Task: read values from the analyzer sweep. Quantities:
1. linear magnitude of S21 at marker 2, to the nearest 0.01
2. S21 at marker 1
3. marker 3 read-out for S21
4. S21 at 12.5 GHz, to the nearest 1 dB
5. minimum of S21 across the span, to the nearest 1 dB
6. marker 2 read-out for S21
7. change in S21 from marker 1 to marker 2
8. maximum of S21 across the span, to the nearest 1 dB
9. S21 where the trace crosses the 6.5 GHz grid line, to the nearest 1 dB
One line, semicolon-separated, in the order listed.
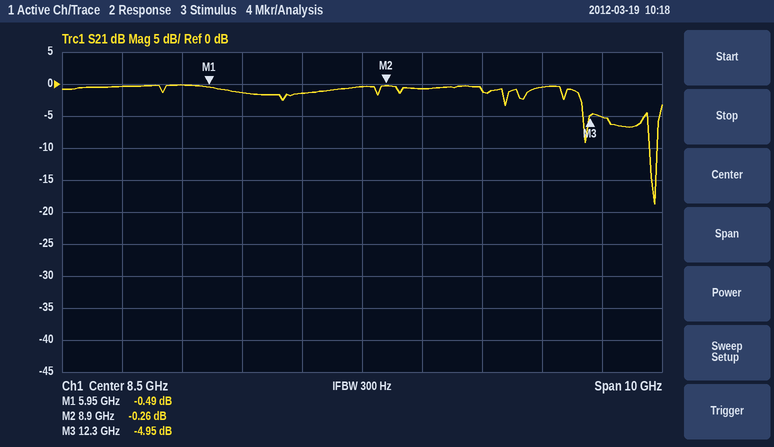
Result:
0.97; -0.49 dB; -4.95 dB; -5 dB; -19 dB; -0.26 dB; 0.23 dB; 0 dB; -1 dB
